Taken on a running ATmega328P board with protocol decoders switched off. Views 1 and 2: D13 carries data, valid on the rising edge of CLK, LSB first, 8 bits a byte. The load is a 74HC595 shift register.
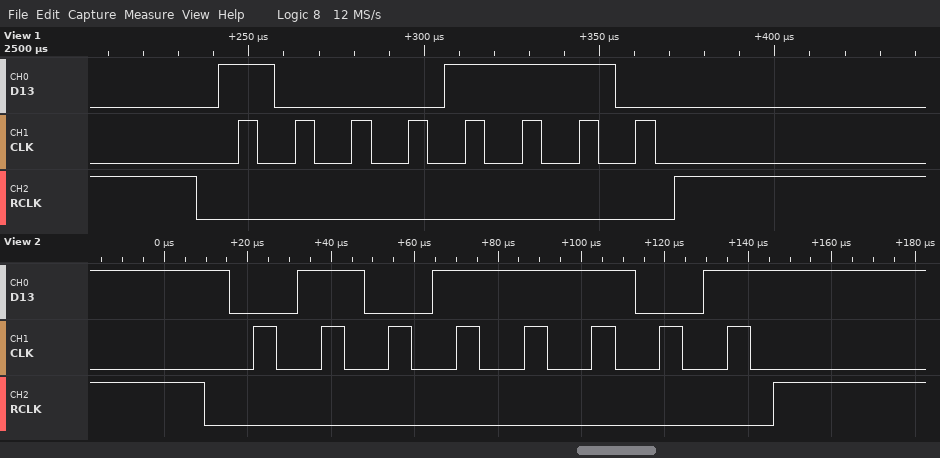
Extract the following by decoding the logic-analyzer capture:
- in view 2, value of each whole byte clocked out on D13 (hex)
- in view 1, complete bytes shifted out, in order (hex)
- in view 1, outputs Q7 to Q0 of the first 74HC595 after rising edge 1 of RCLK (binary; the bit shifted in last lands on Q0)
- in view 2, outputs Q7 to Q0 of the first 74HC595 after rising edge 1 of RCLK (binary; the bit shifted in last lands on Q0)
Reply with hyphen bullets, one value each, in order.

- BA
- 71
- 10001110
- 01011101
